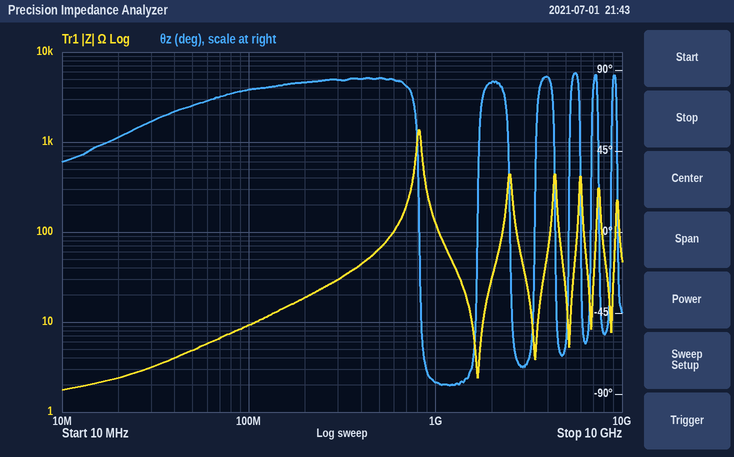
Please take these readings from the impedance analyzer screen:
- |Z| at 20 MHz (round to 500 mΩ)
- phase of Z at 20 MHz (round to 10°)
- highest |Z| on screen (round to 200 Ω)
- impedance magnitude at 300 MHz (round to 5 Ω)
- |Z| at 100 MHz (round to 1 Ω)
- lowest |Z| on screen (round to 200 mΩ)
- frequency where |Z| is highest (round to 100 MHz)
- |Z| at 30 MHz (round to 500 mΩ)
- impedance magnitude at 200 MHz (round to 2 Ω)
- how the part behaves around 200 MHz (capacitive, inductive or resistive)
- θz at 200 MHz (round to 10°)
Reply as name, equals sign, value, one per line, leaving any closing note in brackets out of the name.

|Z| at 20 MHz = 2.5 Ω
phase of Z at 20 MHz = 50°
highest |Z| on screen = 1.4 kΩ
impedance magnitude at 300 MHz = 30 Ω
|Z| at 100 MHz = 9 Ω
lowest |Z| on screen = 1.8 Ω
frequency where |Z| is highest = 800 MHz
|Z| at 30 MHz = 3.0 Ω
impedance magnitude at 200 MHz = 18 Ω
how the part behaves around 200 MHz = inductive
θz at 200 MHz = 80°
